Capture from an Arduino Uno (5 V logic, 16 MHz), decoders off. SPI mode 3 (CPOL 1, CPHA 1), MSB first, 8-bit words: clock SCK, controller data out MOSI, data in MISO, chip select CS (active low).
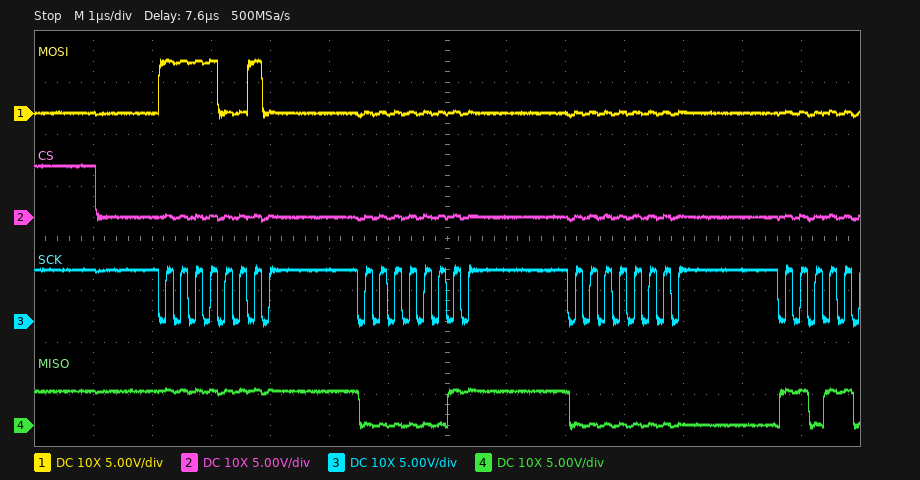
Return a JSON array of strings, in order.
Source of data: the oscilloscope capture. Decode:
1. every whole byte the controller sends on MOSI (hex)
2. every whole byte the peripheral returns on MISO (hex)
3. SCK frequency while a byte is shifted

["F2 00 00", "FF 03 00", "4 MHz"]
